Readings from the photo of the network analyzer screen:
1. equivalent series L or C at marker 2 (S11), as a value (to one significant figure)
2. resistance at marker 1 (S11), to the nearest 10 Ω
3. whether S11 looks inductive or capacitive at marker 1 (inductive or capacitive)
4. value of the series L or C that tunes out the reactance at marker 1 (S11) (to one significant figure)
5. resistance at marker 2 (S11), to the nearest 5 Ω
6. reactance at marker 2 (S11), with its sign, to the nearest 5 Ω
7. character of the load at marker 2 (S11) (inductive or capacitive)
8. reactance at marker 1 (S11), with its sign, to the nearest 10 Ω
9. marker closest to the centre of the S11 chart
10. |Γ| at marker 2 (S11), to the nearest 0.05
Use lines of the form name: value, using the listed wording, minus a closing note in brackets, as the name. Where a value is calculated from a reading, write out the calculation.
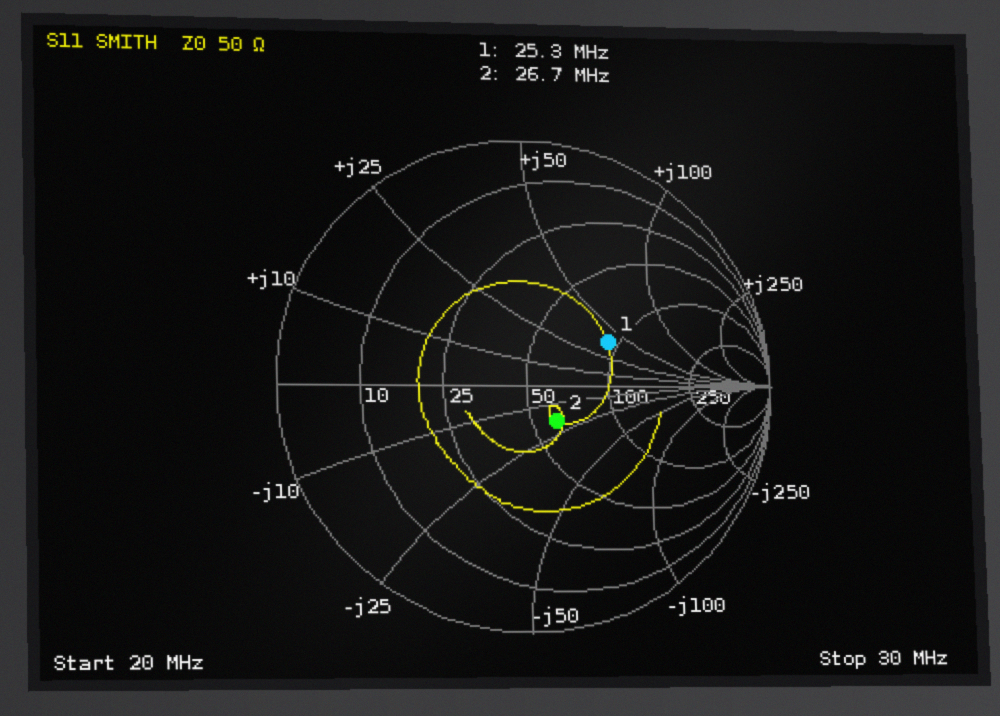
equivalent series L or C at marker 2 (S11), as a value: C = 1/(2π × 26.7 MHz × 20 Ω) ≈ 298 pF, so 300 pF to one significant figure
resistance at marker 1 (S11), to the nearest 10 Ω: 90 Ω
whether S11 looks inductive or capacitive at marker 1: inductive
value of the series L or C that tunes out the reactance at marker 1 (S11): C = 1/(2π × 25.3 MHz × 40 Ω) ≈ 157 pF, so 200 pF to one significant figure
resistance at marker 2 (S11), to the nearest 5 Ω: 60 Ω
reactance at marker 2 (S11), with its sign, to the nearest 5 Ω: -20 Ω
character of the load at marker 2 (S11): capacitive
reactance at marker 1 (S11), with its sign, to the nearest 10 Ω: +40 Ω
marker closest to the centre of the S11 chart: marker 2
|Γ| at marker 2 (S11), to the nearest 0.05: 0.20
